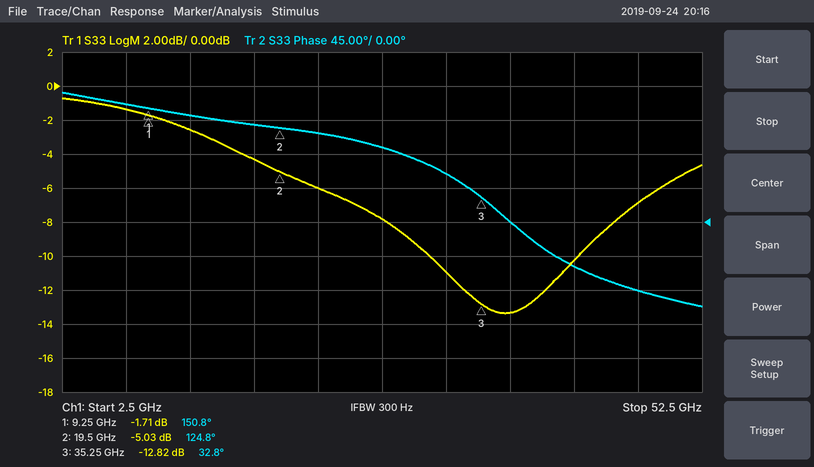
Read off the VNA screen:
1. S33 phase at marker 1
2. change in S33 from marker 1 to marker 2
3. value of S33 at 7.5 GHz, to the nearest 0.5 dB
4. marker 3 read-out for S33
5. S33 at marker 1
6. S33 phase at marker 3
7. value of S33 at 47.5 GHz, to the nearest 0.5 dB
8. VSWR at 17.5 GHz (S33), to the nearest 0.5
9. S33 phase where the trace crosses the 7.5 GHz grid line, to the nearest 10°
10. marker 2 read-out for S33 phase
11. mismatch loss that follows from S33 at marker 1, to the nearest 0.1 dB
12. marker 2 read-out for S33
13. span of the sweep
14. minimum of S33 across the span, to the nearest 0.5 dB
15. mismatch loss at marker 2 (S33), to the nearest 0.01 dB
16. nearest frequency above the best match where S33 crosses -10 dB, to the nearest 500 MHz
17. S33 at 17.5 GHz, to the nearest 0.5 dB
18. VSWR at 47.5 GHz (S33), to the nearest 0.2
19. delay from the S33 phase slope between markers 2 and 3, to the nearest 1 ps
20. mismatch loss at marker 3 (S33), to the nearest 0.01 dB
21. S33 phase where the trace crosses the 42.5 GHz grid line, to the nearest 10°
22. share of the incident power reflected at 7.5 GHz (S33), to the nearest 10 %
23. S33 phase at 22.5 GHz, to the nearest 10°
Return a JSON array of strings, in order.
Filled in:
["150.8°", "-3.32 dB", "-1.5 dB", "-12.82 dB", "-1.71 dB", "32.8°", "-7.0 dB", "4.0", "160°", "124.8°", "4.9 dB", "-5.03 dB", "50 GHz", "-13.5 dB", "1.64 dB", "43.0 GHz", "-4.5 dB", "2.6", "16 ps", "0.23 dB", "-60°", "70 %", "120°"]
